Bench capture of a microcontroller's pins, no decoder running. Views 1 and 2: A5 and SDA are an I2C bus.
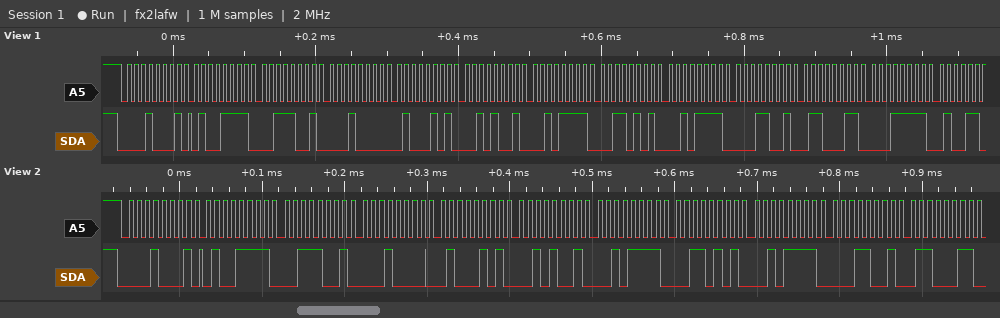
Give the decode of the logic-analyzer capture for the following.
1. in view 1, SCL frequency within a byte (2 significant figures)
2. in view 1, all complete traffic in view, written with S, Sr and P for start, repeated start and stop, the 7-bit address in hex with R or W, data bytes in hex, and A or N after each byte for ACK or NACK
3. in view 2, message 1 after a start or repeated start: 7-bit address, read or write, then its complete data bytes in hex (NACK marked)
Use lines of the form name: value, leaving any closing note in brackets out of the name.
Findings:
in view 1, SCL frequency within a byte: 100 kHz
in view 1, all complete traffic in view, written with S, Sr and P for start, repeated start and stop, the 7-bit address in hex with R or W, data bytes in hex, and A or N after each byte for ACK or NACK: S 08R A 4F A 39 A 10 A 45 A 29 A 2F A 35 A 2F A 19 A 63 A 1F A
in view 2, message 1 after a start or repeated start: 7-bit address, read or write, then its complete data bytes in hex: 0x08 read: 4F 39 10 45 29 2F 35 2F 19 63
